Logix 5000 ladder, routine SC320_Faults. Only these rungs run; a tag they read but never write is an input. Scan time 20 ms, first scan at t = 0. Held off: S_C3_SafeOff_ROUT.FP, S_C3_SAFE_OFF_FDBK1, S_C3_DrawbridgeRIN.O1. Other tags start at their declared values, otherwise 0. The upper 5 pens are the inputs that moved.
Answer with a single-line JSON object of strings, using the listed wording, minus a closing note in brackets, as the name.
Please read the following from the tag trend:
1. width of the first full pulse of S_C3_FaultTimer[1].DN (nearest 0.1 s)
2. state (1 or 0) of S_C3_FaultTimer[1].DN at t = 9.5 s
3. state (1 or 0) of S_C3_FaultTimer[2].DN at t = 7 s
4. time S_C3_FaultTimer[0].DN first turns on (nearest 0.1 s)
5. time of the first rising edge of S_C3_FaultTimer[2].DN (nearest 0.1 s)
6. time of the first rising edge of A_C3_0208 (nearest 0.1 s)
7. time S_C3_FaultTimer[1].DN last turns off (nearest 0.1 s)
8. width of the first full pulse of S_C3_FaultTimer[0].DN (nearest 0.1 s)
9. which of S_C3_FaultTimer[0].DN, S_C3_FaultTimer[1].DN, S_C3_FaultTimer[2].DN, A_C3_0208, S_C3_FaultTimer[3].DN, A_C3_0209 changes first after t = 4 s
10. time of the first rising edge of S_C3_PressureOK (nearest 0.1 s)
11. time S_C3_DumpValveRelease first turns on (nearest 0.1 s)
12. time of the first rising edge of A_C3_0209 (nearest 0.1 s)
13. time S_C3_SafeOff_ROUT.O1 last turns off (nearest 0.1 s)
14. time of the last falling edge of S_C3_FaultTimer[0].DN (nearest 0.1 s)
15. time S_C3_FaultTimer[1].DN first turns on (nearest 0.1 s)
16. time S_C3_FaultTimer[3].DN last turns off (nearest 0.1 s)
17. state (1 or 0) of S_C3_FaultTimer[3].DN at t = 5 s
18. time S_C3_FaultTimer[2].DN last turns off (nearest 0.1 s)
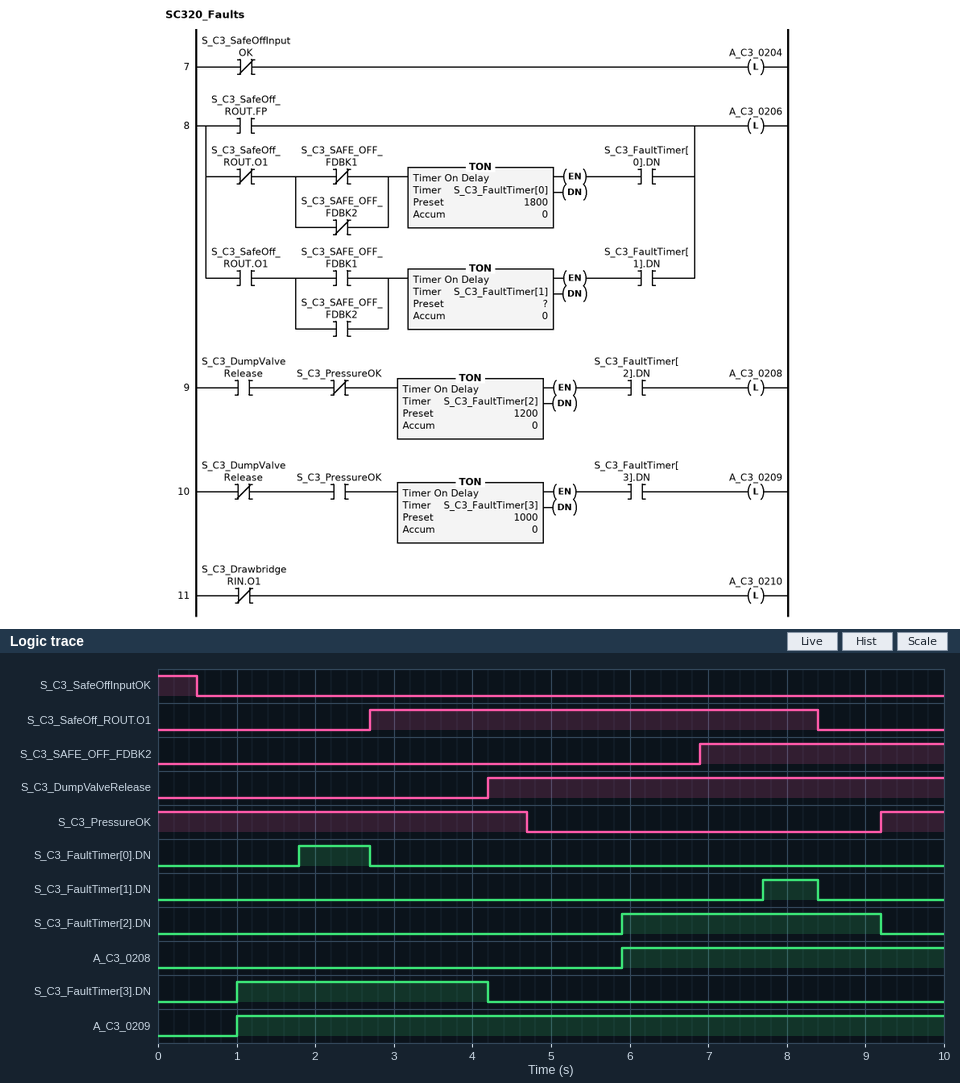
{"width of the first full pulse of S_C3_FaultTimer[1].DN": "0.7 s", "state (1 or 0) of S_C3_FaultTimer[1].DN at t = 9.5 s": "0", "state (1 or 0) of S_C3_FaultTimer[2].DN at t = 7 s": "1", "time S_C3_FaultTimer[0].DN first turns on": "1.8 s", "time of the first rising edge of S_C3_FaultTimer[2].DN": "5.9 s", "time of the first rising edge of A_C3_0208": "5.9 s", "time S_C3_FaultTimer[1].DN last turns off": "8.4 s", "width of the first full pulse of S_C3_FaultTimer[0].DN": "0.9 s", "which of S_C3_FaultTimer[0].DN, S_C3_FaultTimer[1].DN, S_C3_FaultTimer[2].DN, A_C3_0208, S_C3_FaultTimer[3].DN, A_C3_0209 changes first after t = 4 s": "S_C3_FaultTimer[3].DN", "time of the first rising edge of S_C3_PressureOK": "9.2 s", "time S_C3_DumpValveRelease first turns on": "4.2 s", "time of the first rising edge of A_C3_0209": "1.0 s", "time S_C3_SafeOff_ROUT.O1 last turns off": "8.4 s", "time of the last falling edge of S_C3_FaultTimer[0].DN": "2.7 s", "time S_C3_FaultTimer[1].DN first turns on": "7.7 s", "time S_C3_FaultTimer[3].DN last turns off": "4.2 s", "state (1 or 0) of S_C3_FaultTimer[3].DN at t = 5 s": "0", "time S_C3_FaultTimer[2].DN last turns off": "9.2 s"}
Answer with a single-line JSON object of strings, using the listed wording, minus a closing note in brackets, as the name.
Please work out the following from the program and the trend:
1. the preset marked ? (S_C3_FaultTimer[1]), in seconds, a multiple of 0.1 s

{"the preset marked ? (S_C3_FaultTimer[1]), in seconds, a multiple of 0.1 s": "0.8 s"}
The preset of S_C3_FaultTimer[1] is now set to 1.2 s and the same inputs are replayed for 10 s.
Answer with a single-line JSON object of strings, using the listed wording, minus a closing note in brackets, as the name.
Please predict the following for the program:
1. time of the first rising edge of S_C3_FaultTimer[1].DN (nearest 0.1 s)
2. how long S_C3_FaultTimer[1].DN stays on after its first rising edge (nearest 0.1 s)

{"time of the first rising edge of S_C3_FaultTimer[1].DN": "8.1 s", "how long S_C3_FaultTimer[1].DN stays on after its first rising edge": "0.3 s"}
